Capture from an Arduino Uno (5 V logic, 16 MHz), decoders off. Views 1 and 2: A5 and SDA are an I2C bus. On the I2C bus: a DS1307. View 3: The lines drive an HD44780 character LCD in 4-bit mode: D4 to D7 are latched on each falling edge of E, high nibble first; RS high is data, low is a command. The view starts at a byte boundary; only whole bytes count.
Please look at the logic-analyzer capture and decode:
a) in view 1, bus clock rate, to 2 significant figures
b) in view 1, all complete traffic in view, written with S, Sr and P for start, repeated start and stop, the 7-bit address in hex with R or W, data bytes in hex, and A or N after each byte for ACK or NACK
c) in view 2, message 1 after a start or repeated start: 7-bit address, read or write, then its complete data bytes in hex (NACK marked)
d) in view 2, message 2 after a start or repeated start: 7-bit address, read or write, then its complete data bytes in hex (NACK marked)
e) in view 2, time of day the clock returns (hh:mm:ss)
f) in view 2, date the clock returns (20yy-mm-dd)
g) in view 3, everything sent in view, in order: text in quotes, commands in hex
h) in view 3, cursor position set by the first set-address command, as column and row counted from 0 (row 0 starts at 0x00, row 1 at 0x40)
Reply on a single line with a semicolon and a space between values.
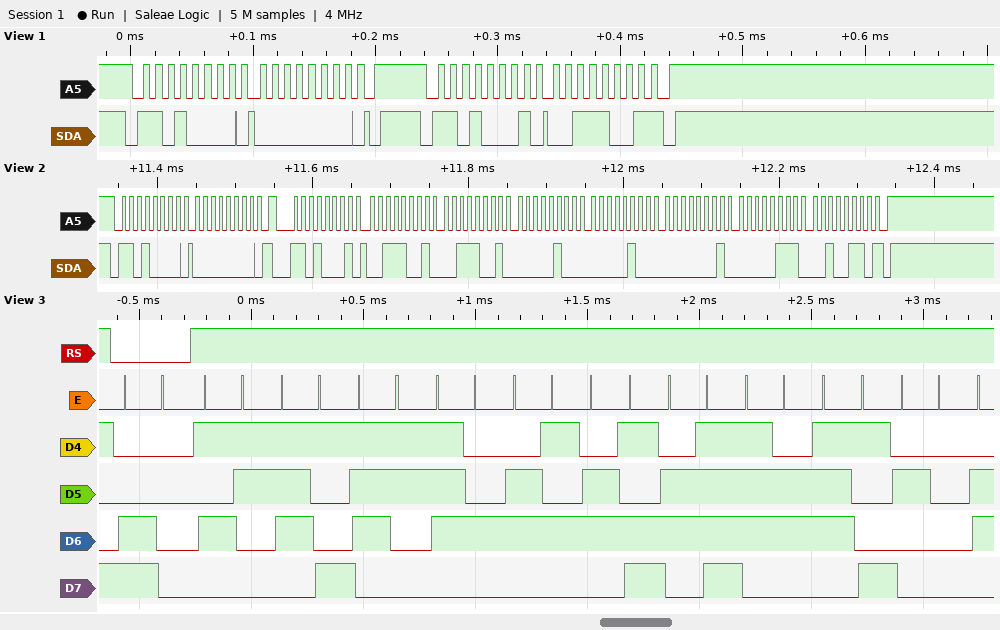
100 kHz; S 68W A 00 A P S 68R A 39 N P; 0x68 write: 00; 0x68 read: 39 39 04 04 01 07 26 NACK; 04:39:39; 2026-07-01; 0xC0 "Systemovy "; column 0, row 1
